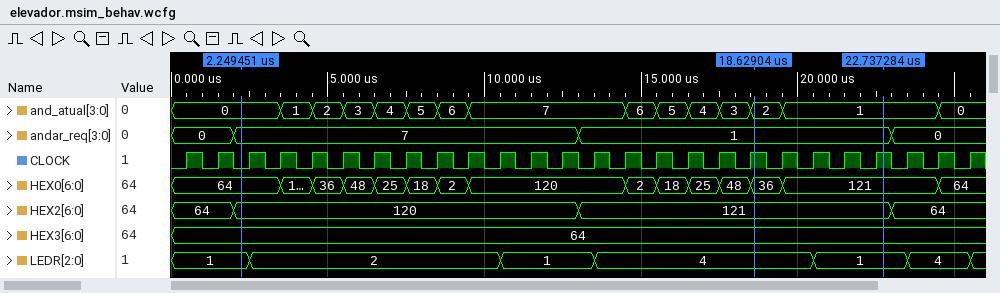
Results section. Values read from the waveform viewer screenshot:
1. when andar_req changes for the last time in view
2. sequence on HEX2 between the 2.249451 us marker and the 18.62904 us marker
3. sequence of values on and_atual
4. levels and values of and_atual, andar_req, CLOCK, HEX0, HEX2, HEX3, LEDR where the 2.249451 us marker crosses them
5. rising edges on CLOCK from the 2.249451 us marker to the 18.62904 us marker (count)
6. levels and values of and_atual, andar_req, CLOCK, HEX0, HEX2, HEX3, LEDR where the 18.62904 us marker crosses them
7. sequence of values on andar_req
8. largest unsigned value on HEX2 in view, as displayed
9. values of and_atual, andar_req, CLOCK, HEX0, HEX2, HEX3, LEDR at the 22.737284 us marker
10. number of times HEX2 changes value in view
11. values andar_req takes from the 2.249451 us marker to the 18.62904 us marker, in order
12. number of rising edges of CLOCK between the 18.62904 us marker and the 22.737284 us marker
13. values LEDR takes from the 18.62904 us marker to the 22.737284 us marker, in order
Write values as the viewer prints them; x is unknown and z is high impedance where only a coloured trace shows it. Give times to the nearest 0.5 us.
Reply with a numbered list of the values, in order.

1. 23 us
2. 120, 121
3. 0, 1, 2, 3, 4, 5, 6, 7, 6, 5, 4, 3, 2, 1, 0
4. and_atual=0, andar_req=7, CLOCK=0, HEX0=64, HEX2=120, HEX3=64, LEDR=1
5. 17
6. and_atual=2, andar_req=1, CLOCK=1, HEX0=36, HEX2=121, HEX3=64, LEDR=4
7. 0, 7, 1, 0
8. 121
9. and_atual=1, andar_req=1, CLOCK=1, HEX0=121, HEX2=121, HEX3=64, LEDR=1
10. 3
11. 7, 1
12. 4
13. 4, 1
